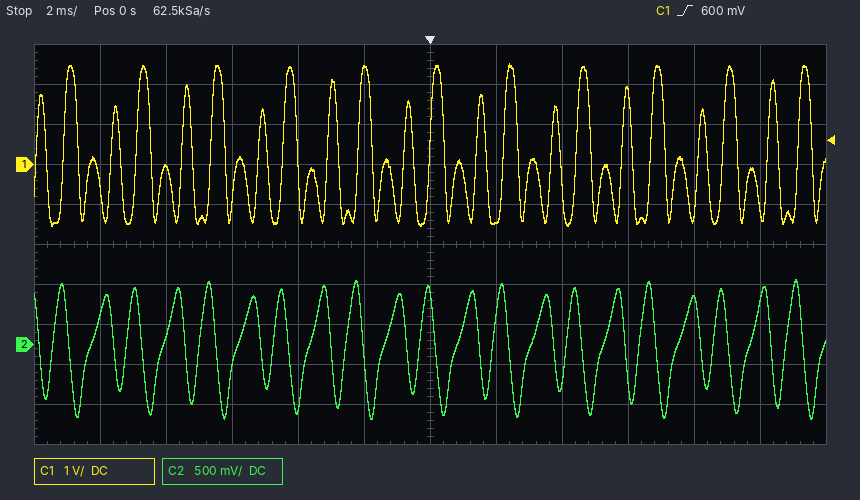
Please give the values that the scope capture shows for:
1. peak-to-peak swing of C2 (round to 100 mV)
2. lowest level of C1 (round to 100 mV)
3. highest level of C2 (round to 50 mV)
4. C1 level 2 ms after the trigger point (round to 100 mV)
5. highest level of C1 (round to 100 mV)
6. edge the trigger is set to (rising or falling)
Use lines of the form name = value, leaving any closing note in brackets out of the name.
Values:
peak-to-peak swing of C2 = 1.70 V
lowest level of C1 = -1.5 V
highest level of C2 = 800 mV
C1 level 2 ms after the trigger point = -1.4 V
highest level of C1 = 2.5 V
edge the trigger is set to = rising
